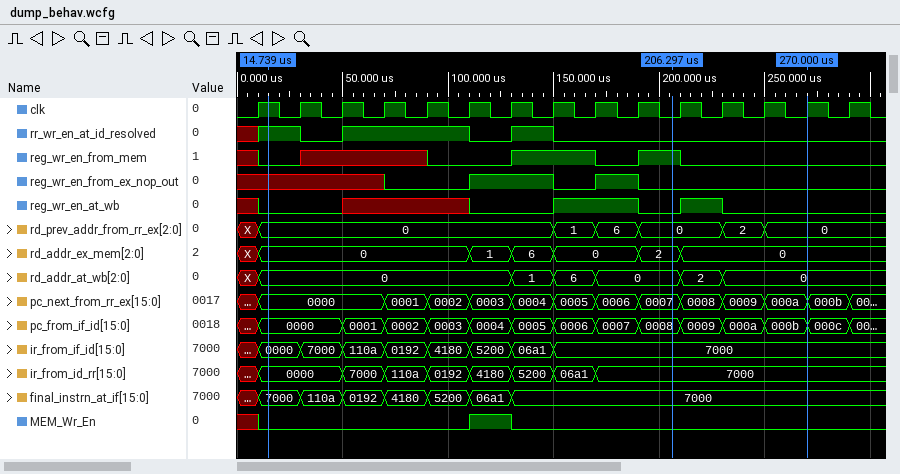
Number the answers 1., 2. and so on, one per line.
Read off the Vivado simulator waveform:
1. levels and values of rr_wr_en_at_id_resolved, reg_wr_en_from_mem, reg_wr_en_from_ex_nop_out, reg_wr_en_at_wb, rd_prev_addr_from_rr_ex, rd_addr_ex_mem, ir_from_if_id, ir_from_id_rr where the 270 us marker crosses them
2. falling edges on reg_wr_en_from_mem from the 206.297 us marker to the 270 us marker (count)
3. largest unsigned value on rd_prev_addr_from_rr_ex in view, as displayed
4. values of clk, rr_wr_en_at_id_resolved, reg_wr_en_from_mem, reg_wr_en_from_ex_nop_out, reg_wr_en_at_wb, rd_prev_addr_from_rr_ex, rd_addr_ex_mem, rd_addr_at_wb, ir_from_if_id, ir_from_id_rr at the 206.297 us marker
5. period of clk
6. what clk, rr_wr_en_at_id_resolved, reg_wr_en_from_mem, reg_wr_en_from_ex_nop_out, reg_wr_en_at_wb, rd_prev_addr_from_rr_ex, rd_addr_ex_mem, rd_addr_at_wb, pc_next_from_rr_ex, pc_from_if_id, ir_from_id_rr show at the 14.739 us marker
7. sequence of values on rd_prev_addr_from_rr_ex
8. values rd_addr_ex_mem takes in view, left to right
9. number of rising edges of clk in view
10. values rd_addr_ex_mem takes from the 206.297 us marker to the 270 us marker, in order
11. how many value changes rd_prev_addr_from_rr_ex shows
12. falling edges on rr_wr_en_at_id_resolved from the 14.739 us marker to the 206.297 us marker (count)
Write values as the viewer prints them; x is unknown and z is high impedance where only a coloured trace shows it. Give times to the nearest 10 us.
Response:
1. rr_wr_en_at_id_resolved=0, reg_wr_en_from_mem=0, reg_wr_en_from_ex_nop_out=0, reg_wr_en_at_wb=0, rd_prev_addr_from_rr_ex=0, rd_addr_ex_mem=0, ir_from_if_id=7000, ir_from_id_rr=7000
2. 1
3. 6
4. clk=0, rr_wr_en_at_id_resolved=0, reg_wr_en_from_mem=1, reg_wr_en_from_ex_nop_out=0, reg_wr_en_at_wb=0, rd_prev_addr_from_rr_ex=0, rd_addr_ex_mem=2, rd_addr_at_wb=0, ir_from_if_id=7000, ir_from_id_rr=7000
5. 20 us
6. clk=1, rr_wr_en_at_id_resolved=1, reg_wr_en_from_mem=0, reg_wr_en_from_ex_nop_out=x, reg_wr_en_at_wb=0, rd_prev_addr_from_rr_ex=0, rd_addr_ex_mem=0, rd_addr_at_wb=0, pc_next_from_rr_ex=0000, pc_from_if_id=0000, ir_from_id_rr=0000
7. X, 0, 1, 6, 0, 2, 0
8. X, 0, 1, 6, 0, 2, 0
9. 15
10. 2, 0
11. 6
12. 3
